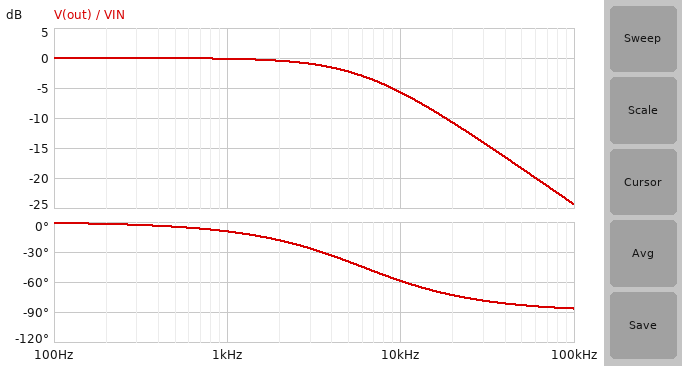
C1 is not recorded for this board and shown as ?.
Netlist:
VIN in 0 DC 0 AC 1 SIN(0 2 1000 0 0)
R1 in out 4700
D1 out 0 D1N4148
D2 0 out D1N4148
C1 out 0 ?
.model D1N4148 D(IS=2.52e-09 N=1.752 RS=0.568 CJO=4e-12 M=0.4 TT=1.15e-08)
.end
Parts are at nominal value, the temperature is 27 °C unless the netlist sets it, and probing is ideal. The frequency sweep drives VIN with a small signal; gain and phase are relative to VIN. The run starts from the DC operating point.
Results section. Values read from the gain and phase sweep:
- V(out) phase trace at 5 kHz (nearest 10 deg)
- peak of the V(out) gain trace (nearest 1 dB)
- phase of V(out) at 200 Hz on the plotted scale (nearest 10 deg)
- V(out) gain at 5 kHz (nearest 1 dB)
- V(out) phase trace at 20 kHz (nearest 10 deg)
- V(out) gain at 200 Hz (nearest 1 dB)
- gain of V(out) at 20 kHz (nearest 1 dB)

-40 deg
0 dB
0 deg
-2 dB
-70 deg
0 dB
-11 dB
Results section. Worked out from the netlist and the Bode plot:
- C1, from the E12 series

5.6 nF
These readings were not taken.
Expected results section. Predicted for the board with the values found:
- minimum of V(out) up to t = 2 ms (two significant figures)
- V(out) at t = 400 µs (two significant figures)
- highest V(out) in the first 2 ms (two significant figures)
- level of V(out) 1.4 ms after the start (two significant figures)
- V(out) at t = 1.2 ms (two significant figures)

-530 mV
500 mV
530 mV
500 mV
530 mV
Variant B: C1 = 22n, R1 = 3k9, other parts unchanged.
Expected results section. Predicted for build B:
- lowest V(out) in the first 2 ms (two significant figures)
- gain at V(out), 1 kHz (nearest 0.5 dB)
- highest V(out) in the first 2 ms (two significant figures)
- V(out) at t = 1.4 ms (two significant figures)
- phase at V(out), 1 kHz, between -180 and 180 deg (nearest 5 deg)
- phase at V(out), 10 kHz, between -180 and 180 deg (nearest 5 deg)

-540 mV
-1.0 dB
540 mV
510 mV
-30 deg
-80 deg
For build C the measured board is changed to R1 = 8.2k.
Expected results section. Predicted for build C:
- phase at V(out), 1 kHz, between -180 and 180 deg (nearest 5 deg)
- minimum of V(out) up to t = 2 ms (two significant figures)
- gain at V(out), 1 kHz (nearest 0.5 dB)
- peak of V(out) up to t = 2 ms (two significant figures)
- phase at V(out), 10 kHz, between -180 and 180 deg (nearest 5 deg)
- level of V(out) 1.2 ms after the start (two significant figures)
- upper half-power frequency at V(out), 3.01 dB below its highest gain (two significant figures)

-15 deg
-510 mV
-0.5 dB
510 mV
-70 deg
500 mV
3.5 kHz
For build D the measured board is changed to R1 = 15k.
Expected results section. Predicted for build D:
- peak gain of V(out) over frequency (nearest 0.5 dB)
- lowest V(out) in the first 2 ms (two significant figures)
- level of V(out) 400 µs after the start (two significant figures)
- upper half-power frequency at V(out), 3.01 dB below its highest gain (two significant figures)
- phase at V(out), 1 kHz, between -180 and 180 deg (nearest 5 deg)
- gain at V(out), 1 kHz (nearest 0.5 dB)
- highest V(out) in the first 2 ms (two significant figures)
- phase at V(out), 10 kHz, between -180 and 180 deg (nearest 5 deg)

0 dB
-480 mV
450 mV
1.9 kHz
-30 deg
-1.0 dB
480 mV
-80 deg
